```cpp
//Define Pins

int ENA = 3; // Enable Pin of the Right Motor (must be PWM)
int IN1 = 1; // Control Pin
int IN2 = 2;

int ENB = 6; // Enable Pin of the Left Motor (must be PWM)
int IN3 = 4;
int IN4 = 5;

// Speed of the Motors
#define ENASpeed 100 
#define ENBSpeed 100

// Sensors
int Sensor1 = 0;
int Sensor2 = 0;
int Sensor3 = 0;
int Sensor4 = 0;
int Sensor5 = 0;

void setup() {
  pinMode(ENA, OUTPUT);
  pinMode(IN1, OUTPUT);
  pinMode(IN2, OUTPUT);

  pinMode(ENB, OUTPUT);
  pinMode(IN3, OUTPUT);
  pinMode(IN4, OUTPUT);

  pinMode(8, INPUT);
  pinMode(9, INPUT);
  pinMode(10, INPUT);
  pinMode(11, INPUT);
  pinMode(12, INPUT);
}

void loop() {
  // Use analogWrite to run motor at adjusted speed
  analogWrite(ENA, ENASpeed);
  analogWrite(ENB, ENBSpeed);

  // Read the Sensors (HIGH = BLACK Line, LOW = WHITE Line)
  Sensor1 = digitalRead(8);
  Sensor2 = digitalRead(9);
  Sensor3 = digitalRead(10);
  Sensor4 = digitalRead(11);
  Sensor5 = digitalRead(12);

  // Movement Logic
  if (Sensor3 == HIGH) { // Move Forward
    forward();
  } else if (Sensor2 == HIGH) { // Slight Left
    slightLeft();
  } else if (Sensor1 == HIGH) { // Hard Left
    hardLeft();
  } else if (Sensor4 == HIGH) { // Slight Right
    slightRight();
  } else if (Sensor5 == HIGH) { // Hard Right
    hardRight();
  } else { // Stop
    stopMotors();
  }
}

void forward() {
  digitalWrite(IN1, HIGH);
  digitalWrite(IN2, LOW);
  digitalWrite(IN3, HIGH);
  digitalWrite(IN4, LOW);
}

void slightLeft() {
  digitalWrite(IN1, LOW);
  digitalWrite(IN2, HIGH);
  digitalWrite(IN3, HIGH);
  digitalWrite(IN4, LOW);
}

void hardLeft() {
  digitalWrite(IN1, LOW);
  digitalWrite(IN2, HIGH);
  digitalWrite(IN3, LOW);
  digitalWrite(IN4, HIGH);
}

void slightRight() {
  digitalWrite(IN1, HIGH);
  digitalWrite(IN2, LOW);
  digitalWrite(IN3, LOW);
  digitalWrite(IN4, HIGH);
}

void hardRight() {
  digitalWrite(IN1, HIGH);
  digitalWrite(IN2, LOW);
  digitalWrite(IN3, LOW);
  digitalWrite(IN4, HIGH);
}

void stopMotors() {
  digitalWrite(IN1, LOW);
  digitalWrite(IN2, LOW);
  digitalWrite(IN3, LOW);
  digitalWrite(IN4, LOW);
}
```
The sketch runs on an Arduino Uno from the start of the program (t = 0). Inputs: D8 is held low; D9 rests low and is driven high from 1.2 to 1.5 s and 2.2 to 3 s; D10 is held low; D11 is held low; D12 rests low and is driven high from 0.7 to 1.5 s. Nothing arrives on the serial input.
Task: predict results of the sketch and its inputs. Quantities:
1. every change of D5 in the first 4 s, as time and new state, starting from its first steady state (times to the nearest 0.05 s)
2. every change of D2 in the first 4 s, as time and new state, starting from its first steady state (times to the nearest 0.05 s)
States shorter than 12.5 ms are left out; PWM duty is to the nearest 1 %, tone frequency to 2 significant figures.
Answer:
0 s low; 0.7 s high; 1.2 s low
0 s low; 1.2 s high; 1.5 s low; 2.2 s high; 3 s low
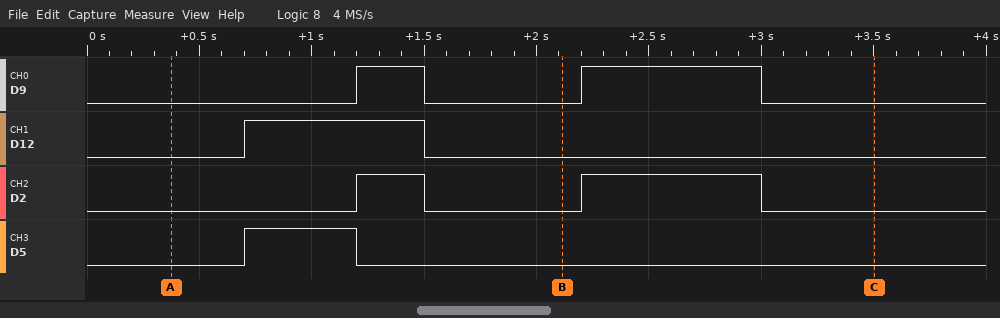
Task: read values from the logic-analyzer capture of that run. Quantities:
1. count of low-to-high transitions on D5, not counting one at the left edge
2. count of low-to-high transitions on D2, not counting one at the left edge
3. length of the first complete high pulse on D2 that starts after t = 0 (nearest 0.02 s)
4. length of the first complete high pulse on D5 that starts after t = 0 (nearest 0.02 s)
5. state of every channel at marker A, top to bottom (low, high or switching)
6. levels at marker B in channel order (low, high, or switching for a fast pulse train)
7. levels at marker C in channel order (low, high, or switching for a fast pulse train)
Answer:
1
2
0.30 s
0.50 s
D9 low, D12 low, D2 low, D5 low
D9 low, D12 low, D2 low, D5 low
D9 low, D12 low, D2 low, D5 low
